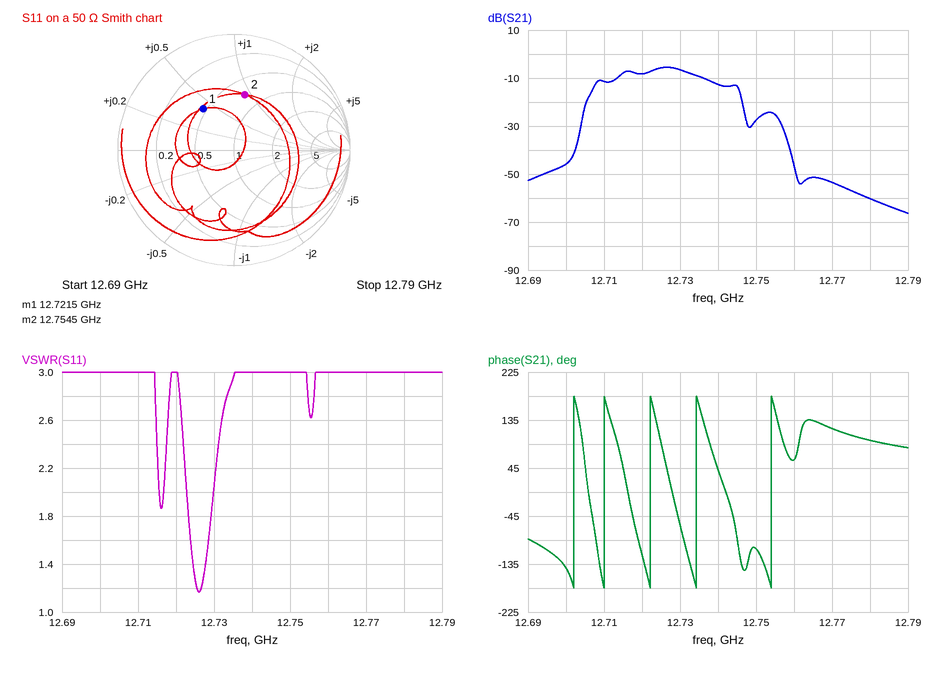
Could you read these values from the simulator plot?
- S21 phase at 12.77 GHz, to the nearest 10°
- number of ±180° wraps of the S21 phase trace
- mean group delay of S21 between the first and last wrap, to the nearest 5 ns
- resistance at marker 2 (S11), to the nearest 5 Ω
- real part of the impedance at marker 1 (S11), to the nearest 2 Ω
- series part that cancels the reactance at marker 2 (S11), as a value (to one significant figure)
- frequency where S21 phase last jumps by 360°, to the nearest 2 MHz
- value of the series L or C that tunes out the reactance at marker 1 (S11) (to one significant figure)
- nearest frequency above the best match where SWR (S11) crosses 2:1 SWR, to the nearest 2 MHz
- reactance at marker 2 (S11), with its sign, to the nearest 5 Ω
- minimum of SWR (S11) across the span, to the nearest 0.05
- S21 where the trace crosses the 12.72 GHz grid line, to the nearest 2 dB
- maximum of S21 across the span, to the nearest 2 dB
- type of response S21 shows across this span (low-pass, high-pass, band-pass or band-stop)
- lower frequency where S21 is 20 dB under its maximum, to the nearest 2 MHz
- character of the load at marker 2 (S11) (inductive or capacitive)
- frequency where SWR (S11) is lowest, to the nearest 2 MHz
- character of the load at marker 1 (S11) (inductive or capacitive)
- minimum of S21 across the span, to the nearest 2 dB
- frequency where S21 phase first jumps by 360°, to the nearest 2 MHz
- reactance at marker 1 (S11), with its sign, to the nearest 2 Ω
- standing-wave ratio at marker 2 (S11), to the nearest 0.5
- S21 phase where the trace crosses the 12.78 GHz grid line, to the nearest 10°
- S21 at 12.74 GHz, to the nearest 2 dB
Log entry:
120°
5
75 ns
35 Ω
24 Ω
300 fF
12.754 GHz
600 fF
12.730 GHz
+45 Ω
1.15
-8 dB
-6 dB
band-pass
12.704 GHz
inductive
12.726 GHz
inductive
-66 dB
12.702 GHz
+20 Ω
3.0
100°
-12 dB
